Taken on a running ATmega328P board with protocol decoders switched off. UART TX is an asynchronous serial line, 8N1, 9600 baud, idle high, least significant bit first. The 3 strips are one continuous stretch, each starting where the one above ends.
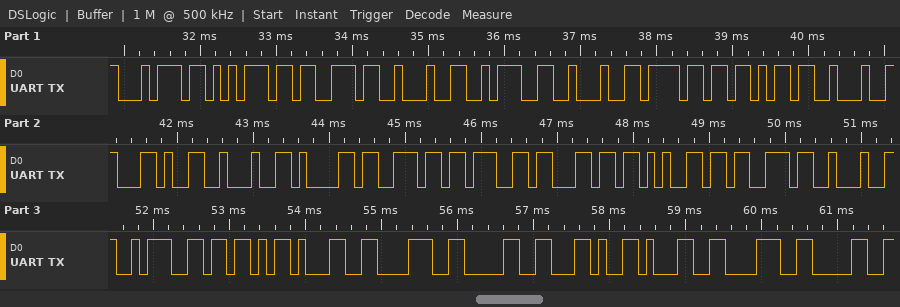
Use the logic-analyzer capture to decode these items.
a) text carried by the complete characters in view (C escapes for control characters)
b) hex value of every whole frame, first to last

"tus\":\"ok\",\"angles\":[180,180"
74 75 73 22 3A 22 6F 6B 22 2C 22 61 6E 67 6C 65 73 22 3A 5B 31 38 30 2C 31 38 30
